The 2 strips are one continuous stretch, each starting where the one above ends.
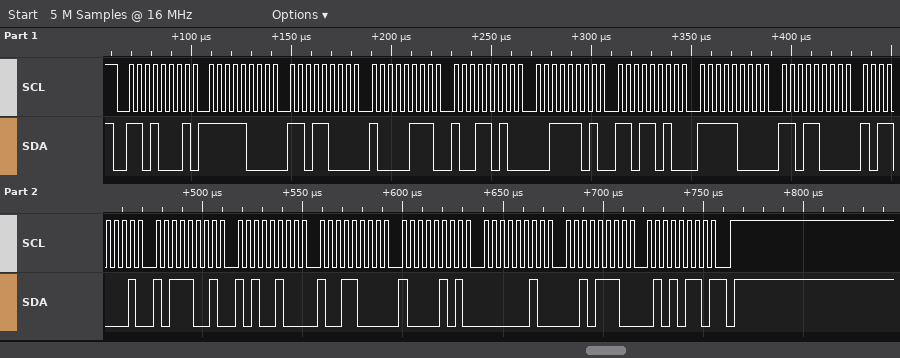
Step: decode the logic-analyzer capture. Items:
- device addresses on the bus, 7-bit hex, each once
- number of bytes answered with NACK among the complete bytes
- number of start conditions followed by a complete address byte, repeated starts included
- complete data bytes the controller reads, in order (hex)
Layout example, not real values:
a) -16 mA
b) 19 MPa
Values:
a) 0x68
b) 1
c) 1
d) F8 D8 87 9A 3D DA F8 D8 B1 B9 A4 98 85 02 2E 56
